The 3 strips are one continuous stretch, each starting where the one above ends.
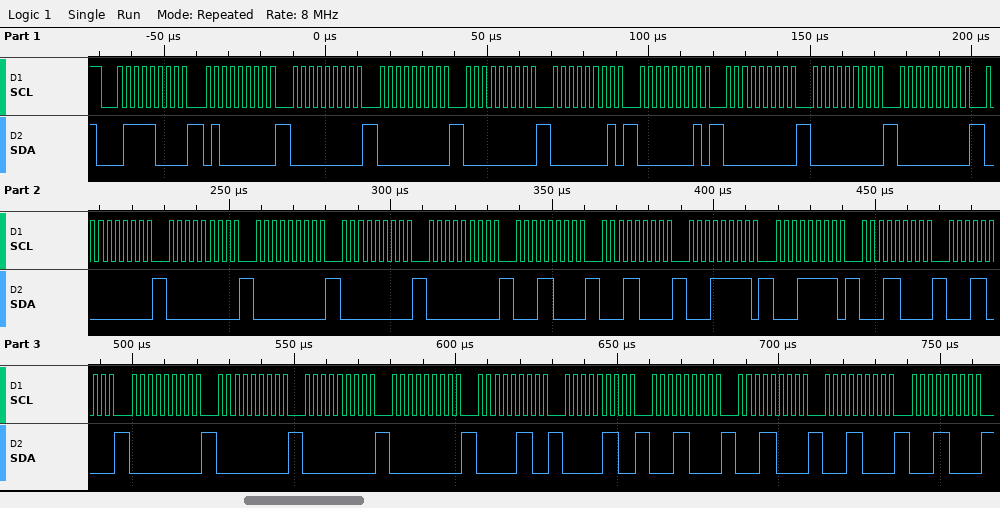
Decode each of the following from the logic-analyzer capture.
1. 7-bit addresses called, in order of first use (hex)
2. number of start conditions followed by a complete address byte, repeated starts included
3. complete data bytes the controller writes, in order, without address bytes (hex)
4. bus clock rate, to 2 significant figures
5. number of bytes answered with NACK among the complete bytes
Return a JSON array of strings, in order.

["0x3C", "1", "40 00 00 00 01 01 00 00 00 00 00 00 00 00 18 18 1F 1F 18 18 00 00 00 00 06 06 18 18 18 18", "400 kHz", "0"]
